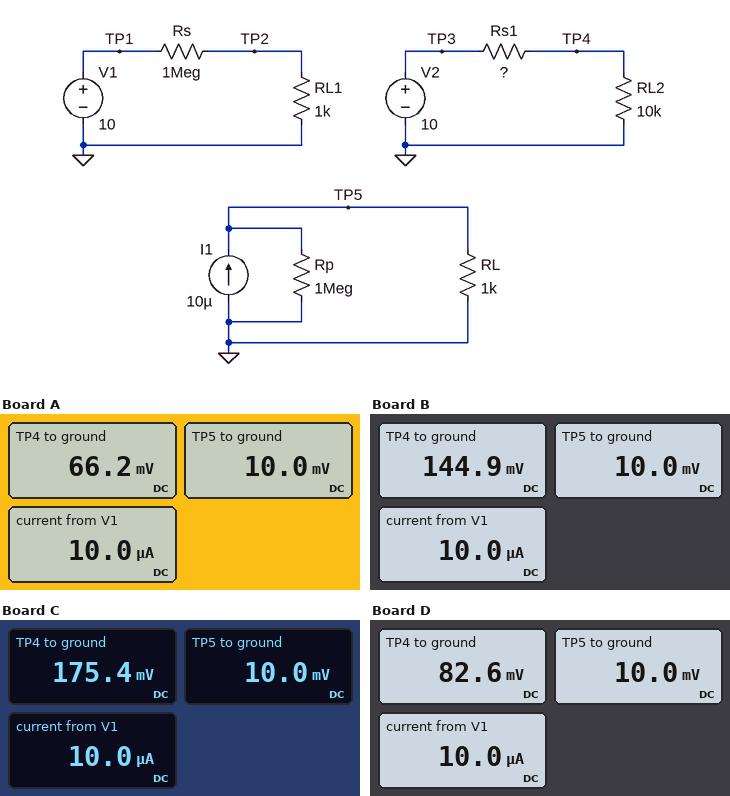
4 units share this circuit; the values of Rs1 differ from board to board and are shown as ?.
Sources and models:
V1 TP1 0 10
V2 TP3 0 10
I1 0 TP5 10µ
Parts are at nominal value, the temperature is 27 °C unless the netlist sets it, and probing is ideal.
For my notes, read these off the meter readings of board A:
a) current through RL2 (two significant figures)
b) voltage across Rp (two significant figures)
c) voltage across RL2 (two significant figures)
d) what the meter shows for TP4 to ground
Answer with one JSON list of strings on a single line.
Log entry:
["6.6 µA", "10 mV", "66 mV", "66.2 mV"]
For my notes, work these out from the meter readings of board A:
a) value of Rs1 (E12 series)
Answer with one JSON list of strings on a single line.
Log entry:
["1.5 MΩ"]
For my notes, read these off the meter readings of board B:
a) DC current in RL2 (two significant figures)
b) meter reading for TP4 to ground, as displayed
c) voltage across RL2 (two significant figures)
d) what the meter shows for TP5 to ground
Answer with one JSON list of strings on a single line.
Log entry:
["14 µA", "144.9 mV", "140 mV", "10.0 mV"]
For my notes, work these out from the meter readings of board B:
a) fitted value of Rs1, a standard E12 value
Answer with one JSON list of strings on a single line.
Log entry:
["680 kΩ"]
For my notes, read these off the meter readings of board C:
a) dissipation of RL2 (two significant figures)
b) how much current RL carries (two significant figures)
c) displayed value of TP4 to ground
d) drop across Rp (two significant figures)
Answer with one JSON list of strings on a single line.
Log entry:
["3.1 µW", "10 µA", "175.4 mV", "10 mV"]
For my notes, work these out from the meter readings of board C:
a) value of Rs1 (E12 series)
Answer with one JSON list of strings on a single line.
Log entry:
["560 kΩ"]
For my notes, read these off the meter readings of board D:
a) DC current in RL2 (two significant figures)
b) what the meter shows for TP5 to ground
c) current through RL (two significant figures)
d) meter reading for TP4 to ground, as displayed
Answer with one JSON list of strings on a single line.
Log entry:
["8.3 µA", "10.0 mV", "10 µA", "82.6 mV"]
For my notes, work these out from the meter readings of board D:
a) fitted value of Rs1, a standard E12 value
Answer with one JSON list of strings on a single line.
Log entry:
["1.2 MΩ"]
